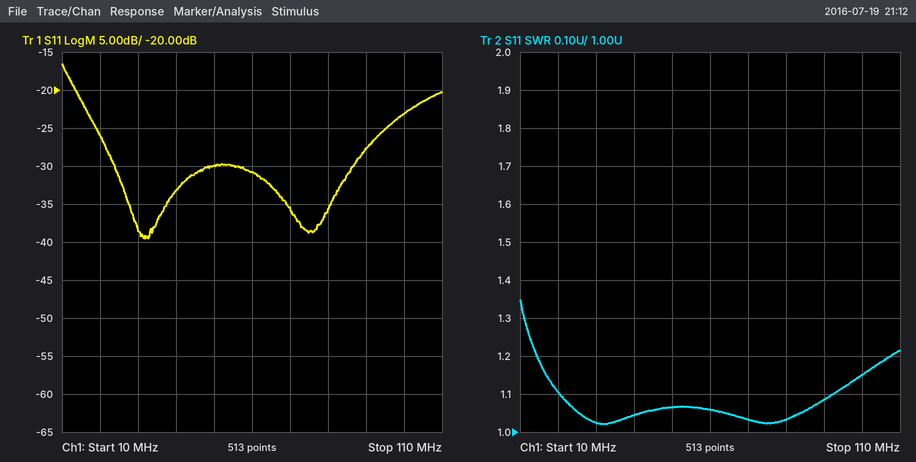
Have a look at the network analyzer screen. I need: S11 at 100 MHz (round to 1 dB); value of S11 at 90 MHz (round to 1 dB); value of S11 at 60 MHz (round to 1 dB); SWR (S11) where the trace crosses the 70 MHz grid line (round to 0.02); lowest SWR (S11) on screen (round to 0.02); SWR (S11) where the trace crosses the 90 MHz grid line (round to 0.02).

-23 dB
-28 dB
-31 dB
1.04
1.02
1.08
